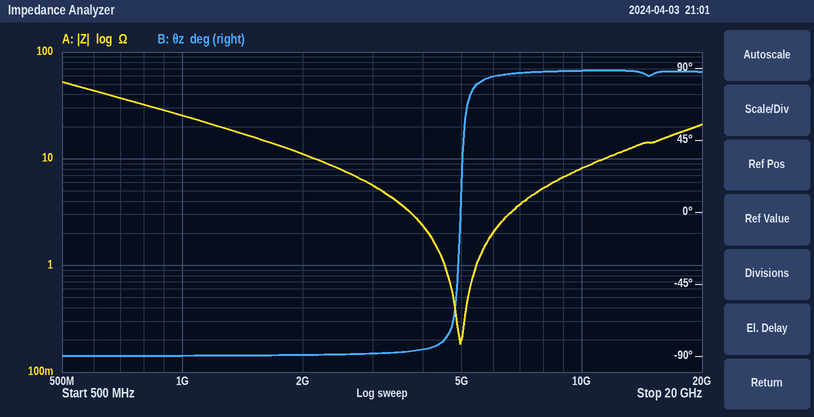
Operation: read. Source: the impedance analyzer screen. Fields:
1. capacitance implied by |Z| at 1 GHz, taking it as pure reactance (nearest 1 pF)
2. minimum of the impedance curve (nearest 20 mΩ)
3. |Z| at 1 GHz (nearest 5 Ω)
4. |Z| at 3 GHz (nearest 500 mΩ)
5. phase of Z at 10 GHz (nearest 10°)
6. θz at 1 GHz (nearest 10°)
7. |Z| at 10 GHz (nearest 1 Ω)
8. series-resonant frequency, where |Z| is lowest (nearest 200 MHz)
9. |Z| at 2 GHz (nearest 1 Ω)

6 pF
180 mΩ
25 Ω
5.5 Ω
90°
-90°
8 Ω
5.0 GHz
11 Ω
